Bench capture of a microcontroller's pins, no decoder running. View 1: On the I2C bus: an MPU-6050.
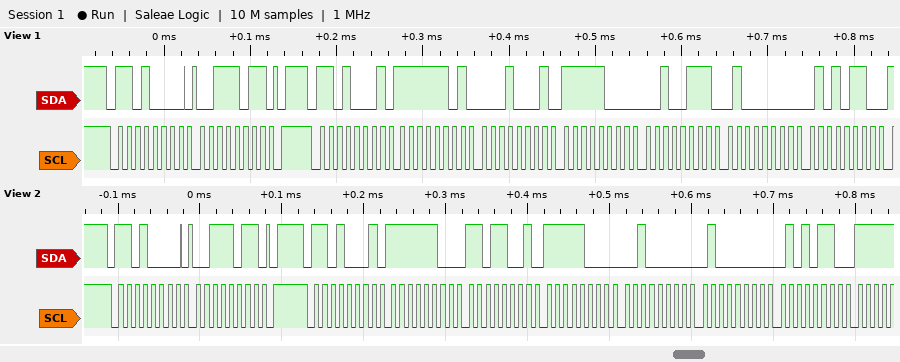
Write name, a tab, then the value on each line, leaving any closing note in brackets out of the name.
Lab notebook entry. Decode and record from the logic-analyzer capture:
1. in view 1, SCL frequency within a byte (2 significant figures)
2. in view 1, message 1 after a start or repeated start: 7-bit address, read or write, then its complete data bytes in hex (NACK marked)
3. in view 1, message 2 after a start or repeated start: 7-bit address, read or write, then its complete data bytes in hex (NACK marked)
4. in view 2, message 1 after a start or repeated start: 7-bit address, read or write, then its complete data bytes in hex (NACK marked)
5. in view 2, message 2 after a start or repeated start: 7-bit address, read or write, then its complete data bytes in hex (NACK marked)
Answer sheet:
in view 1, SCL frequency within a byte	100 kHz
in view 1, message 1 after a start or repeated start: 7-bit address, read or write, then its complete data bytes in hex	0x68 write: 3B
in view 1, message 2 after a start or repeated start: 7-bit address, read or write, then its complete data bytes in hex	0x68 read: FD 11 F8 27 40 56
in view 2, message 1 after a start or repeated start: 7-bit address, read or write, then its complete data bytes in hex	0x68 write: 3B
in view 2, message 2 after a start or repeated start: 7-bit address, read or write, then its complete data bytes in hex	0x68 read: FC D9 F8 20 40 56
